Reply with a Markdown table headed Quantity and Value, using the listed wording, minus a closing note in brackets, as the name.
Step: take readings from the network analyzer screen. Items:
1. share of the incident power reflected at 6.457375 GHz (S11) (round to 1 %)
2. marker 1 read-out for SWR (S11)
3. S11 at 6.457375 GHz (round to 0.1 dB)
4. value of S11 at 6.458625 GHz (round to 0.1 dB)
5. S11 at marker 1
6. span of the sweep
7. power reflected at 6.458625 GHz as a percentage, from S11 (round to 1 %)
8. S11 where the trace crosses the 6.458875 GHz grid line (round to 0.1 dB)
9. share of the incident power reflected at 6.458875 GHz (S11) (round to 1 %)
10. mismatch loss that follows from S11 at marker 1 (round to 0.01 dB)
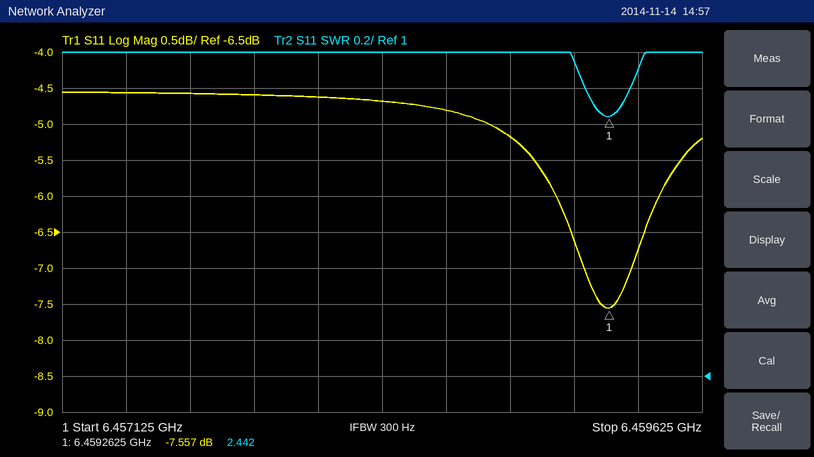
| Quantity | Value |
|---|---|
| share of the incident power reflected at 6.457375 GHz (S11) | 35 % |
| marker 1 read-out for SWR | 2.442 |
| S11 at 6.457375 GHz | -4.6 dB |
| value of S11 at 6.458625 GHz | -4.8 dB |
| S11 at marker 1 | -7.557 dB |
| span of the sweep | 2.5 MHz |
| power reflected at 6.458625 GHz as a percentage, from S11 | 33 % |
| S11 where the trace crosses the 6.458875 GHz grid line | -5.2 dB |
| share of the incident power reflected at 6.458875 GHz (S11) | 30 % |
| mismatch loss that follows from S11 at marker 1 | 0.84 dB |
